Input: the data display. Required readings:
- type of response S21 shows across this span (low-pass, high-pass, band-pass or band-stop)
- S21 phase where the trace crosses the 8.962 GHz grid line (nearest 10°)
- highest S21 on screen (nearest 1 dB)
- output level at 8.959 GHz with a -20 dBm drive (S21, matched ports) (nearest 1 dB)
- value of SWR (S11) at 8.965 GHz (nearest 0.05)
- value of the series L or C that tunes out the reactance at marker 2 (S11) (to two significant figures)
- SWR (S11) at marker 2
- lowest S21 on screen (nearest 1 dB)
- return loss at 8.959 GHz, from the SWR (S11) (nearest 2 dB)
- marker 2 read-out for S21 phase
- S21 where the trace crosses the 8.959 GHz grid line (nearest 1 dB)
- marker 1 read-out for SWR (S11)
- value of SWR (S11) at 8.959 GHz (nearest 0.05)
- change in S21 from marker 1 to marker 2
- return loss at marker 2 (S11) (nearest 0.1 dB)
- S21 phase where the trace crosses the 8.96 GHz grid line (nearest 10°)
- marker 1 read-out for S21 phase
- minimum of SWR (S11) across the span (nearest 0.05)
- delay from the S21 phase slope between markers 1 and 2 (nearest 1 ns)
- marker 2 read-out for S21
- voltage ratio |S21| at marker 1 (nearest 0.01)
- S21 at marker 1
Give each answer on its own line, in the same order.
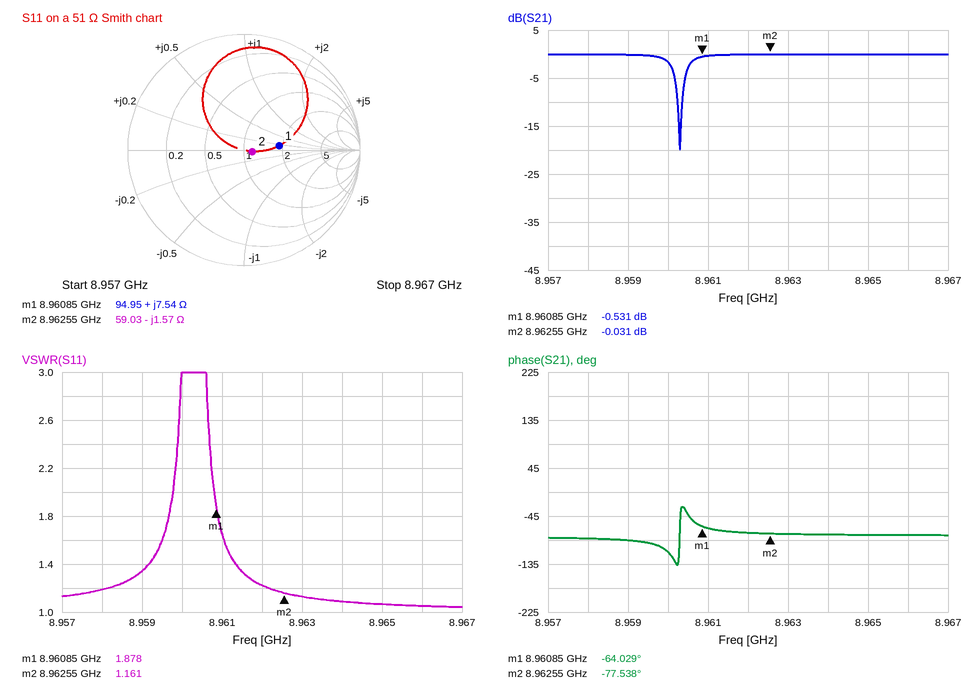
band-stop
-80°
0 dB
-20 dBm
1.05
28 pH
1.161
-20 dB
16 dB
-77.538°
0 dB
1.878
1.35
0.500 dB
22.6 dB
-110°
-64.029°
1.05
22 ns
-0.031 dB
0.94
-0.531 dB
